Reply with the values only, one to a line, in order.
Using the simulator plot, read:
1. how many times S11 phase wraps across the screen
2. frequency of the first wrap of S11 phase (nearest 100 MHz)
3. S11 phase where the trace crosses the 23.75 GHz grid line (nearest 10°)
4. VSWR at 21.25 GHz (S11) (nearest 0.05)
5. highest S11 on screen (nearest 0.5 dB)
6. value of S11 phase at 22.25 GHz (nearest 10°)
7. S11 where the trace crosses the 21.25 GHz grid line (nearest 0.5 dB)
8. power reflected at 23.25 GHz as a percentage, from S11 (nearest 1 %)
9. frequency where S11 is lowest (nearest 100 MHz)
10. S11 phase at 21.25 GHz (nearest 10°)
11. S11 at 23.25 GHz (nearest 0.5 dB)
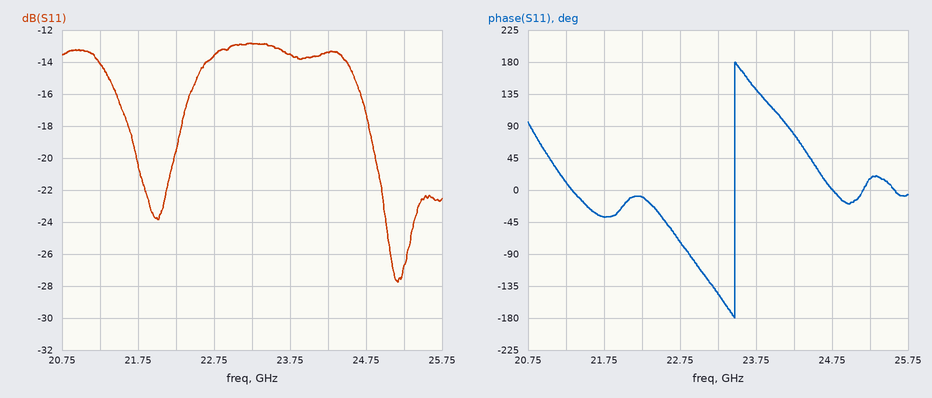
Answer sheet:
1
23.5 GHz
140°
1.50
-13.0 dB
-10°
-14.0 dB
5 %
25.2 GHz
10°
-13.0 dB
